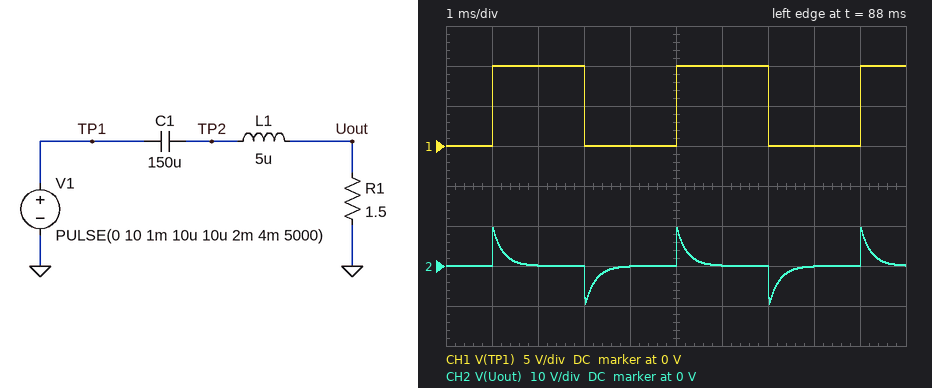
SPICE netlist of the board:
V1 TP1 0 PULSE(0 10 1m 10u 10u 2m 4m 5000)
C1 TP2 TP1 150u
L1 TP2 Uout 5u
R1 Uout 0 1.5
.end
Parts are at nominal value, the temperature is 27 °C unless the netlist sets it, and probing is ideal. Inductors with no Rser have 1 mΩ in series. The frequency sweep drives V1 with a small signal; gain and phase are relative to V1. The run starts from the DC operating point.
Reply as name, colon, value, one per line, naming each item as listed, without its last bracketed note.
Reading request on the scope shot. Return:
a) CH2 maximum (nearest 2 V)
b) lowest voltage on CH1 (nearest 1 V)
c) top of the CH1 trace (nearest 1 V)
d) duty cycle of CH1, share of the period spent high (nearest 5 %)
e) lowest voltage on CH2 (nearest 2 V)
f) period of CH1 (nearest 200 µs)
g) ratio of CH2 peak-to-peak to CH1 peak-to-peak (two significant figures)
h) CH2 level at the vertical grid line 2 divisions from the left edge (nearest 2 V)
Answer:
CH2 maximum: 10 V
lowest voltage on CH1: 0 V
top of the CH1 trace: 10 V
duty cycle of CH1, share of the period spent high: 50 %
lowest voltage on CH2: -10 V
period of CH1: 4.0 ms
ratio of CH2 peak-to-peak to CH1 peak-to-peak: 1.9
CH2 level at the vertical grid line 2 divisions from the left edge: 0 V
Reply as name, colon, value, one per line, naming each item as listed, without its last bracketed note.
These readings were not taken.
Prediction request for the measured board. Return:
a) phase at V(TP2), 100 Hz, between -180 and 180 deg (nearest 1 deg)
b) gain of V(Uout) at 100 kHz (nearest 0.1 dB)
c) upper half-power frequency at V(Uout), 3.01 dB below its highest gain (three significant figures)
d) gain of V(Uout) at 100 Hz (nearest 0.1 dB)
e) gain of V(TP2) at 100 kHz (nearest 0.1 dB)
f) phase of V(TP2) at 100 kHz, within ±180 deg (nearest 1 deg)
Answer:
phase at V(TP2), 100 Hz, between -180 and 180 deg: 82 deg
gain of V(Uout) at 100 kHz: -7.3 dB
upper half-power frequency at V(Uout), 3.01 dB below its highest gain: 48.5 kHz
gain of V(Uout) at 100 Hz: -17.1 dB
gain of V(TP2) at 100 kHz: 0 dB
phase of V(TP2) at 100 kHz, within ±180 deg: 0 deg
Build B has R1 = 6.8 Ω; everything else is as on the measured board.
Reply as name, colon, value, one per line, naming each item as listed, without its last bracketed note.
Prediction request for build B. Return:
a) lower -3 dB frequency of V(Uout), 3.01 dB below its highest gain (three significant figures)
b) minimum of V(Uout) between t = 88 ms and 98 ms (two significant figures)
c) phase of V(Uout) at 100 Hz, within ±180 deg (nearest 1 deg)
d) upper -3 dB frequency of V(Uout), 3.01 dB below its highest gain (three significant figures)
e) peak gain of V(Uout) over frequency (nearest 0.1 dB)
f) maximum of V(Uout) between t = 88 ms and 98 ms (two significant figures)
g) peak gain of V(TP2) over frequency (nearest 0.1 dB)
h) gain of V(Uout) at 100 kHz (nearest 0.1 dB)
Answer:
lower -3 dB frequency of V(Uout), 3.01 dB below its highest gain: 156 Hz
minimum of V(Uout) between t = 88 ms and 98 ms: -8.7 V
phase of V(Uout) at 100 Hz, within ±180 deg: 57 deg
upper -3 dB frequency of V(Uout), 3.01 dB below its highest gain: 217 kHz
peak gain of V(Uout) over frequency: 0 dB
maximum of V(Uout) between t = 88 ms and 98 ms: 8.7 V
peak gain of V(TP2) over frequency: 0 dB
gain of V(Uout) at 100 kHz: -0.8 dB
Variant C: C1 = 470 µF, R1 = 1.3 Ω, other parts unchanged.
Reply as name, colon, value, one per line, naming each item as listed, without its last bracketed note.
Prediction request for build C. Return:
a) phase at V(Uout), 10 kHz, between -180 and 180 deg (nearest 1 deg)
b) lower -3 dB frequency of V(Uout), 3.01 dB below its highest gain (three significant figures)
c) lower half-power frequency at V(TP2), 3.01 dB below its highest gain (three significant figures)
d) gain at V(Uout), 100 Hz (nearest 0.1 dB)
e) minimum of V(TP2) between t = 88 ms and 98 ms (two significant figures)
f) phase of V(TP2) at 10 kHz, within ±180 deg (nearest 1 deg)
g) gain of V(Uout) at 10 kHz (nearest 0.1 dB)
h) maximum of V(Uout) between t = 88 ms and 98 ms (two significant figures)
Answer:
phase at V(Uout), 10 kHz, between -180 and 180 deg: -12 deg
lower -3 dB frequency of V(Uout), 3.01 dB below its highest gain: 259 Hz
lower half-power frequency at V(TP2), 3.01 dB below its highest gain: 262 Hz
gain at V(Uout), 100 Hz: -8.9 dB
minimum of V(TP2) between t = 88 ms and 98 ms: -9.6 V
phase of V(TP2) at 10 kHz, within ±180 deg: 1 deg
gain of V(Uout) at 10 kHz: -0.2 dB
maximum of V(Uout) between t = 88 ms and 98 ms: 9.4 V
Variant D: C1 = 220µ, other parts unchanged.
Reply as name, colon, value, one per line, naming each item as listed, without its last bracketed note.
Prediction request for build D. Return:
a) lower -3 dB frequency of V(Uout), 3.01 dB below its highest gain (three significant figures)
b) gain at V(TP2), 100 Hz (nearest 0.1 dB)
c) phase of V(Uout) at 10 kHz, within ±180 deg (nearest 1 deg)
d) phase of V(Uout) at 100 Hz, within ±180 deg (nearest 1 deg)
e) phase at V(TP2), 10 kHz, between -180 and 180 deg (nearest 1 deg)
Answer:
lower -3 dB frequency of V(Uout), 3.01 dB below its highest gain: 477 Hz
gain at V(TP2), 100 Hz: -13.8 dB
phase of V(Uout) at 10 kHz, within ±180 deg: -9 deg
phase of V(Uout) at 100 Hz, within ±180 deg: 78 deg
phase at V(TP2), 10 kHz, between -180 and 180 deg: 3 deg
